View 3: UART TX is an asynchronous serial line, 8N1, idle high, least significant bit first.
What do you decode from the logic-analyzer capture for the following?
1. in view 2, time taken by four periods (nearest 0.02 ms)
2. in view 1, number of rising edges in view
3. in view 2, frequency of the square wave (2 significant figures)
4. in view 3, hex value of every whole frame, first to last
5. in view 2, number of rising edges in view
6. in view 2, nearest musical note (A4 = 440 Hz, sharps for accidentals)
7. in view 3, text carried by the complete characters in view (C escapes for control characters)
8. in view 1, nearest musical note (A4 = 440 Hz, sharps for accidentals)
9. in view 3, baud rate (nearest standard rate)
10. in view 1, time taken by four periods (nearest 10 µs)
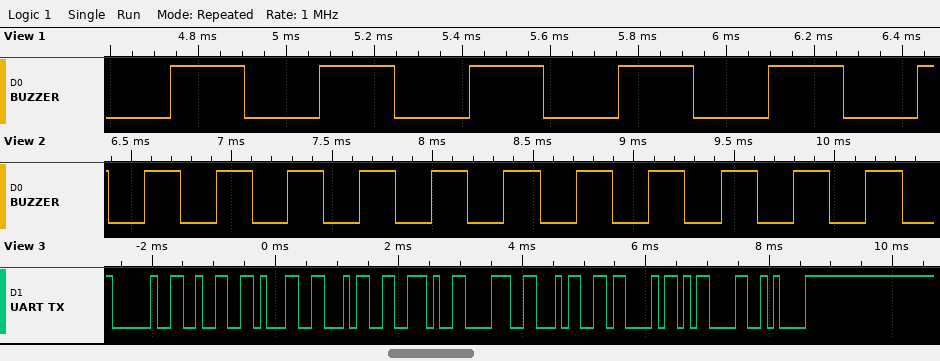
1.44 ms
6
2.8 kHz
20 32 31 34 2E 38 34 43 0D 0A
11
F7
" 214.84C\r\n"
F#7
9600 baud
1350 µs
